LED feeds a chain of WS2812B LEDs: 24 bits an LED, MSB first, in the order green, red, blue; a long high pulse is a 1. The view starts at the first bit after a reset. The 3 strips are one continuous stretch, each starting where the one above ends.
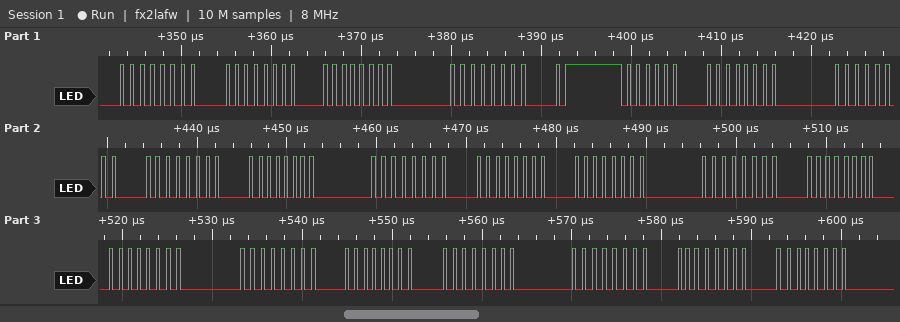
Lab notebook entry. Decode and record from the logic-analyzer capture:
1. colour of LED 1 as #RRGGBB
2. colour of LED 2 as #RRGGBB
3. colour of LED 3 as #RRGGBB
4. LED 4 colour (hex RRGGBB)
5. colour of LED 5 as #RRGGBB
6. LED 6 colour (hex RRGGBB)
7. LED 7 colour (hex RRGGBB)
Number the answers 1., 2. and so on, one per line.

1. #000000
2. #400000
3. #000000
4. #000000
5. #000000
6. #000000
7. #000000
